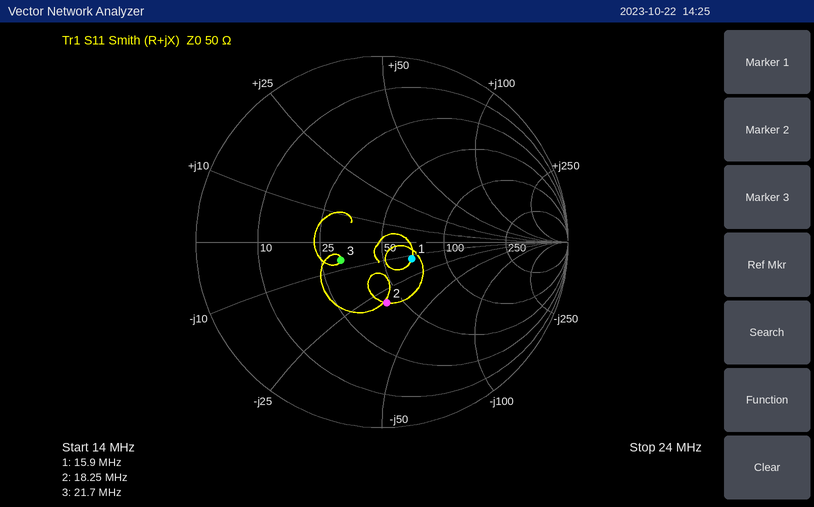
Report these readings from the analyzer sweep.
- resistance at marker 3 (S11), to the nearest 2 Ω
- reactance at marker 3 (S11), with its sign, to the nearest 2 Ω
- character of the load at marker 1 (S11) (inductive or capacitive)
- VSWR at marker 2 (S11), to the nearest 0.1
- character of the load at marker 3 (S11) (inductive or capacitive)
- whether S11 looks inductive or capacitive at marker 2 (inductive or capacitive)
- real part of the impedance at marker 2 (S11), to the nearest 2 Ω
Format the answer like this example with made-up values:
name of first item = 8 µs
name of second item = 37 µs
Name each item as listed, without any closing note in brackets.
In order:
resistance at marker 3 (S11), to the nearest 2 Ω = 32 Ω
reactance at marker 3 (S11), with its sign, to the nearest 2 Ω = -6 Ω
character of the load at marker 1 (S11) = capacitive
VSWR at marker 2 (S11), to the nearest 0.1 = 2.0
character of the load at marker 3 (S11) = capacitive
whether S11 looks inductive or capacitive at marker 2 = capacitive
real part of the impedance at marker 2 (S11), to the nearest 2 Ω = 42 Ω
